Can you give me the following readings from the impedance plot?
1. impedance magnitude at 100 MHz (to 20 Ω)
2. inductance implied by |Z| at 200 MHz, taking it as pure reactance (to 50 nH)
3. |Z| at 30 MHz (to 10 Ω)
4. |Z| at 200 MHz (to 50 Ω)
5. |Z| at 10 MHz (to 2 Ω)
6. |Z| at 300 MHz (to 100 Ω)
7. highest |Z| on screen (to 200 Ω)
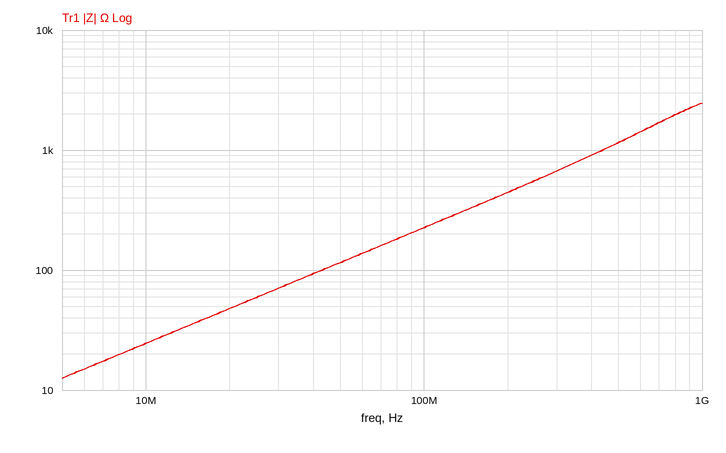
220 Ω
350 nH
70 Ω
450 Ω
24 Ω
700 Ω
2.4 kΩ
